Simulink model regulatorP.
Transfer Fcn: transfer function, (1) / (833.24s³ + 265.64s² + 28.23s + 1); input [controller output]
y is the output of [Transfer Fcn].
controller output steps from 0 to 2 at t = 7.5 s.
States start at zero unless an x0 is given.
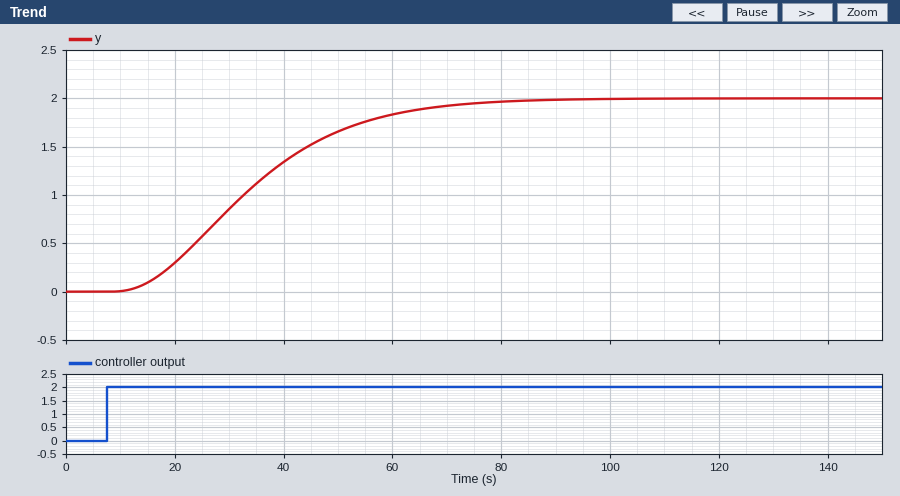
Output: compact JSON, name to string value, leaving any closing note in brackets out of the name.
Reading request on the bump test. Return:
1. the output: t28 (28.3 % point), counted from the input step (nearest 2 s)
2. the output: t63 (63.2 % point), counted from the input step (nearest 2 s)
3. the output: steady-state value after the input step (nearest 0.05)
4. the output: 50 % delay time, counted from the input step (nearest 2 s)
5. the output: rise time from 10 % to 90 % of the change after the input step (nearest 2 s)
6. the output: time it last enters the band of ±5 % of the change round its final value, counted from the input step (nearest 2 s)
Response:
{"the output: t28 (28.3 % point), counted from the input step": "18 s", "the output: t63 (63.2 % point), counted from the input step": "30 s", "the output: steady-state value after the input step": "2.00", "the output: 50 % delay time, counted from the input step": "26 s", "the output: rise time from 10 % to 90 % of the change after the input step": "40 s", "the output: time it last enters the band of ±5 % of the change round its final value, counted from the input step": "60 s"}
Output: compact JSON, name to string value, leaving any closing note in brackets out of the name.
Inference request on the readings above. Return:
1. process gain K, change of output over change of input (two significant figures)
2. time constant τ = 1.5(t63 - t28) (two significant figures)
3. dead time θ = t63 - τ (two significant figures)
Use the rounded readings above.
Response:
{"process gain K, change of output over change of input": "1.0", "time constant τ = 1.5(t63 - t28)": "18 s", "dead time θ = t63 - τ": "12 s"}
